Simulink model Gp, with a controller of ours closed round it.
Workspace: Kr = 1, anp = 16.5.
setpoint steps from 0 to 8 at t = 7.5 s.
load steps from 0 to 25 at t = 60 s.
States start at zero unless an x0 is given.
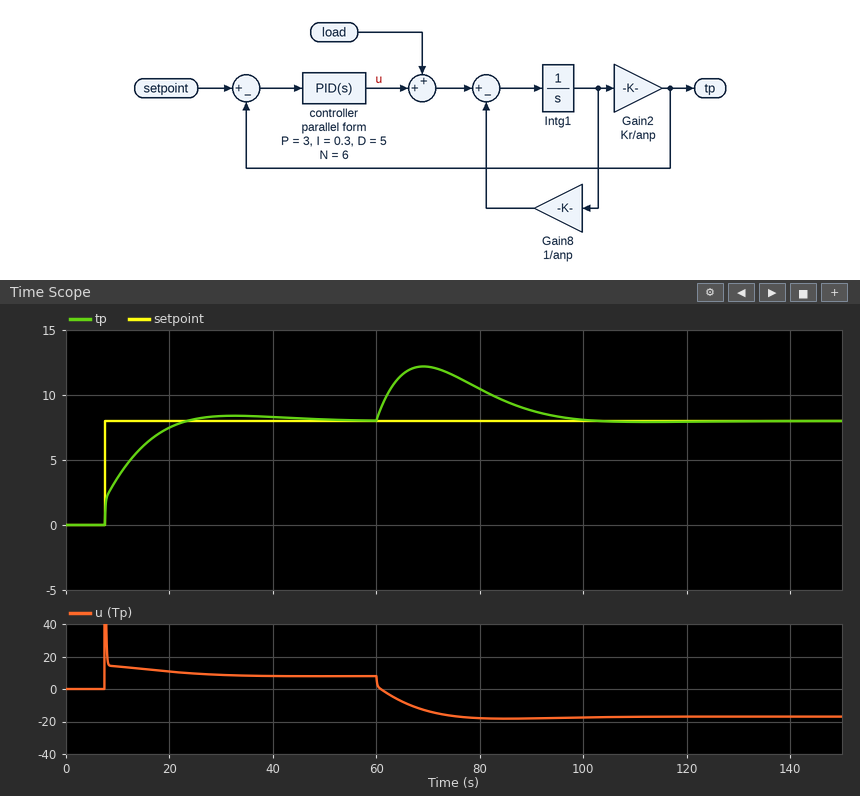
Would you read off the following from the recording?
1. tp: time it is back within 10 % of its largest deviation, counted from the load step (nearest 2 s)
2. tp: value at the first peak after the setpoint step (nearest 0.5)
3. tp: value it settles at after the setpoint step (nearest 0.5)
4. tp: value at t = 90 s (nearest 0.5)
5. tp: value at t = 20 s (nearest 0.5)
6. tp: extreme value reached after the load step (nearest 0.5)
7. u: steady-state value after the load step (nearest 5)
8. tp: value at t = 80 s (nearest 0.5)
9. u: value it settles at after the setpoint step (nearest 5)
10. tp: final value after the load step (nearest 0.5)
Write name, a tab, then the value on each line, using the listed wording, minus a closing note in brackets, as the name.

tp: time it is back within 10 % of its largest deviation, counted from the load step	34 s
tp: value at the first peak after the setpoint step	8.5
tp: value it settles at after the setpoint step	8.0
tp: value at t = 90 s	9.0
tp: value at t = 20 s	7.5
tp: extreme value reached after the load step	12.0
u: steady-state value after the load step	-15
tp: value at t = 80 s	10.5
u: value it settles at after the setpoint step	10
tp: final value after the load step	8.0
